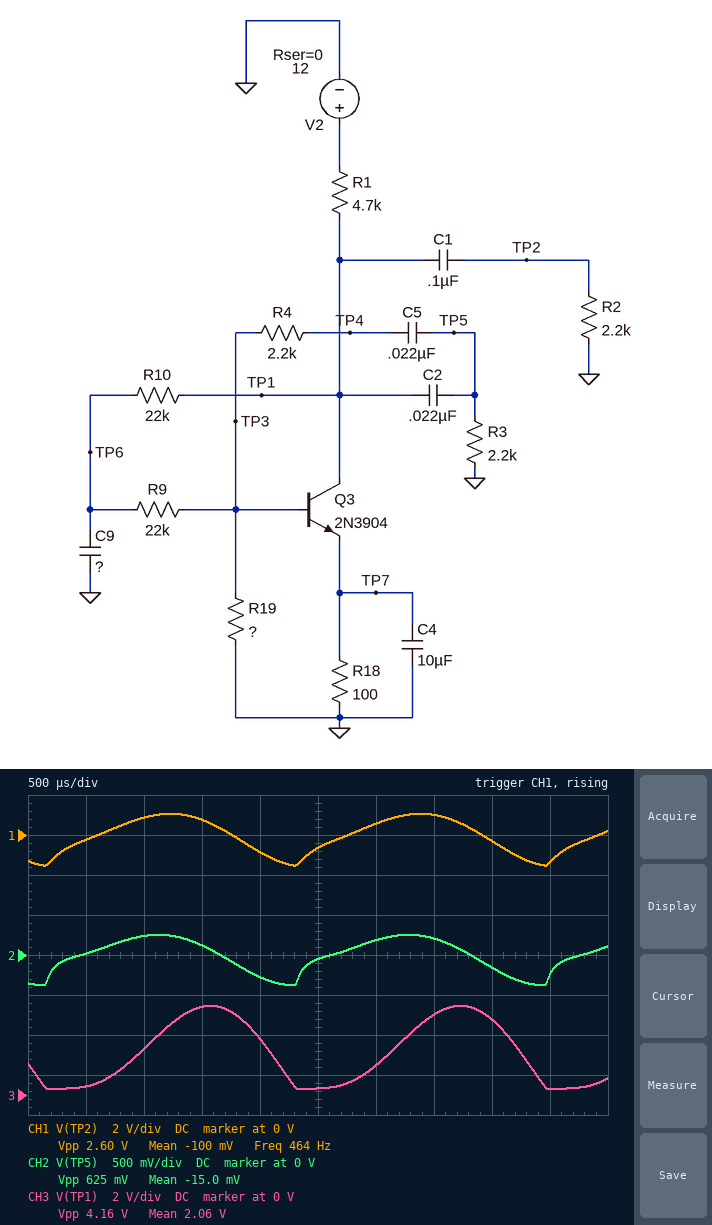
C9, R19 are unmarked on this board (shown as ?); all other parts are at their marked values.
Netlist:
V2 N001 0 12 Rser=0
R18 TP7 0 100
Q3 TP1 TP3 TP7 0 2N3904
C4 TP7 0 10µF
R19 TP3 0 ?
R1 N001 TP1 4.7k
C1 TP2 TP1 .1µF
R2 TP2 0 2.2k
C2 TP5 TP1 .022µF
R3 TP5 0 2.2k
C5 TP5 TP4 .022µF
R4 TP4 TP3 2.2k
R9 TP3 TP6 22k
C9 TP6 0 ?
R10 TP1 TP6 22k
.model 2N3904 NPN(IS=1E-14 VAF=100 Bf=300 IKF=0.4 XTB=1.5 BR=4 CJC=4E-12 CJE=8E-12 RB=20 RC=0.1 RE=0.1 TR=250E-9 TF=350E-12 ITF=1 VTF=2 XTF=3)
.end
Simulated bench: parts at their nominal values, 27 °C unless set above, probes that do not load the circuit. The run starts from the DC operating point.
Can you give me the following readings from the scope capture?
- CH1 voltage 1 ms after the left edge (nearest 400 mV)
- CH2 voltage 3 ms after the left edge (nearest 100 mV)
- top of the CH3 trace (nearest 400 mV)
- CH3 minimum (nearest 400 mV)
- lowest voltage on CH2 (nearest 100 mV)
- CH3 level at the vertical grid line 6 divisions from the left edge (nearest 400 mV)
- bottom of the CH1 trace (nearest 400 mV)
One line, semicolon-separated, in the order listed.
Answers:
800 mV; 200 mV; 4.4 V; 400 mV; -400 mV; 1.6 V; -1.6 V
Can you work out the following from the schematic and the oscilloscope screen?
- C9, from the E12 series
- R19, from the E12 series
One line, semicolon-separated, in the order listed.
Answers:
100 nF; 39 kΩ
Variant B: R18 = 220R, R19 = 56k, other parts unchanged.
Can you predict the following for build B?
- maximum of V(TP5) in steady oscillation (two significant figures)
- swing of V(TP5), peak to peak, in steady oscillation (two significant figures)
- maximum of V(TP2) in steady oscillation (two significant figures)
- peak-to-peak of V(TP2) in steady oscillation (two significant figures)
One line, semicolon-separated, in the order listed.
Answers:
240 mV; 610 mV; 1.0 V; 2.5 V
